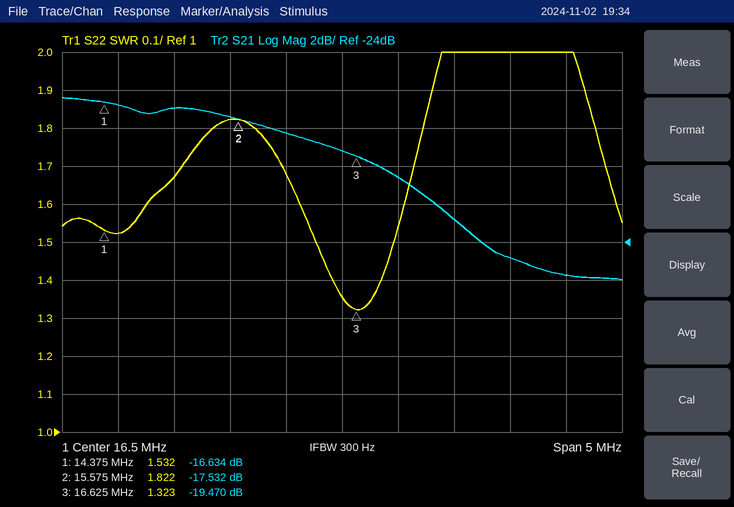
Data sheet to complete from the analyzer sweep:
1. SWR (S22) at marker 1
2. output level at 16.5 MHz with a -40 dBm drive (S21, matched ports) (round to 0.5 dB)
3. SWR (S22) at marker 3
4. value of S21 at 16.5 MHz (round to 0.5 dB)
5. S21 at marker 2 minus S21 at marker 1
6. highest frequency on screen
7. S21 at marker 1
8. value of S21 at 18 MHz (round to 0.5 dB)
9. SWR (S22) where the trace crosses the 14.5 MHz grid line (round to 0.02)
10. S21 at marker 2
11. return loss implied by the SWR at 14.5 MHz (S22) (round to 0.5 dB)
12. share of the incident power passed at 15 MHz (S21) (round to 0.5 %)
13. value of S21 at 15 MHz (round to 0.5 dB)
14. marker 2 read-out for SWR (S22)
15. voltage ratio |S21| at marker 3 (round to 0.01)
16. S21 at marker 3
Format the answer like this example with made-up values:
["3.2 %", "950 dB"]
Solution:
["1.532", "-59.0 dBm", "1.323", "-19.0 dB", "-0.898 dB", "19 MHz", "-16.634 dB", "-25.0 dB", "1.52", "-17.532 dB", "13.5 dB", "2.0 %", "-17.0 dB", "1.822", "0.11", "-19.470 dB"]
